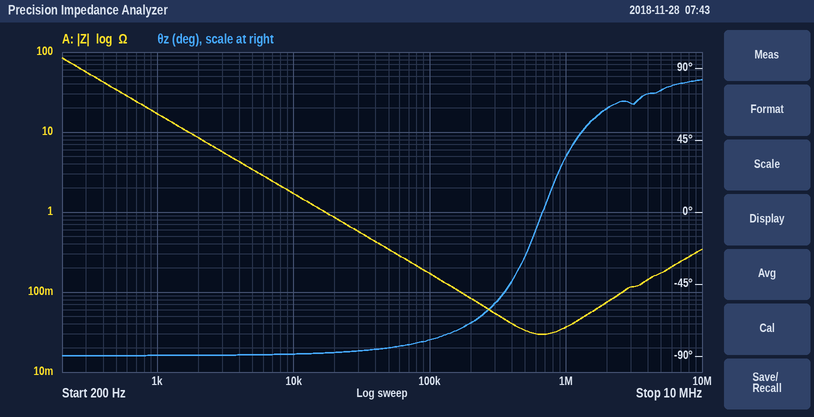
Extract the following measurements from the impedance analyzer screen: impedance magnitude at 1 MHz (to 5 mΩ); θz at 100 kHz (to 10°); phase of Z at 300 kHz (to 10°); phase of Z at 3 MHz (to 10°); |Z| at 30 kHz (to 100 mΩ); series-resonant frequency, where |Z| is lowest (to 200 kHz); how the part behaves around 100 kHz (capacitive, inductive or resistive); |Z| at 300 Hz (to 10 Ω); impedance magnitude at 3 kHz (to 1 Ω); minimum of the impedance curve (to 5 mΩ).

35 mΩ
-80°
-60°
70°
600 mΩ
600 kHz
capacitive
60 Ω
6 Ω
30 mΩ
